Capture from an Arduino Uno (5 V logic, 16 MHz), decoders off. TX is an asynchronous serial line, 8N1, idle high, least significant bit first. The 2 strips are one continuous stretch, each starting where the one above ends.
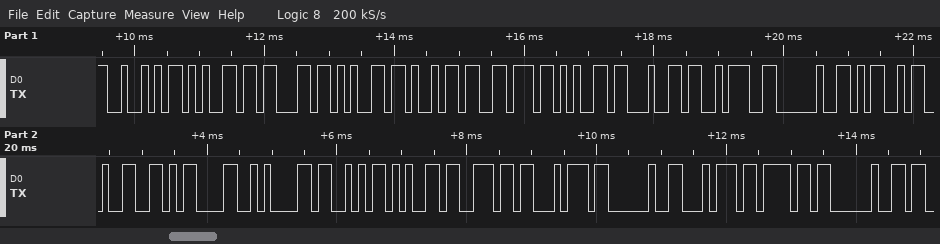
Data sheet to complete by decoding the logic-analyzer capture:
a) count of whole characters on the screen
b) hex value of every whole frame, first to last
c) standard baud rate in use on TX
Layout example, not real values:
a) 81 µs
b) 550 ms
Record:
a) 22
b) 52 65 63 65 69 76 65 64 3A 20 4D 32 0D 0A 53 65 6E 74 20 74 6F 20
c) 9600 baud
